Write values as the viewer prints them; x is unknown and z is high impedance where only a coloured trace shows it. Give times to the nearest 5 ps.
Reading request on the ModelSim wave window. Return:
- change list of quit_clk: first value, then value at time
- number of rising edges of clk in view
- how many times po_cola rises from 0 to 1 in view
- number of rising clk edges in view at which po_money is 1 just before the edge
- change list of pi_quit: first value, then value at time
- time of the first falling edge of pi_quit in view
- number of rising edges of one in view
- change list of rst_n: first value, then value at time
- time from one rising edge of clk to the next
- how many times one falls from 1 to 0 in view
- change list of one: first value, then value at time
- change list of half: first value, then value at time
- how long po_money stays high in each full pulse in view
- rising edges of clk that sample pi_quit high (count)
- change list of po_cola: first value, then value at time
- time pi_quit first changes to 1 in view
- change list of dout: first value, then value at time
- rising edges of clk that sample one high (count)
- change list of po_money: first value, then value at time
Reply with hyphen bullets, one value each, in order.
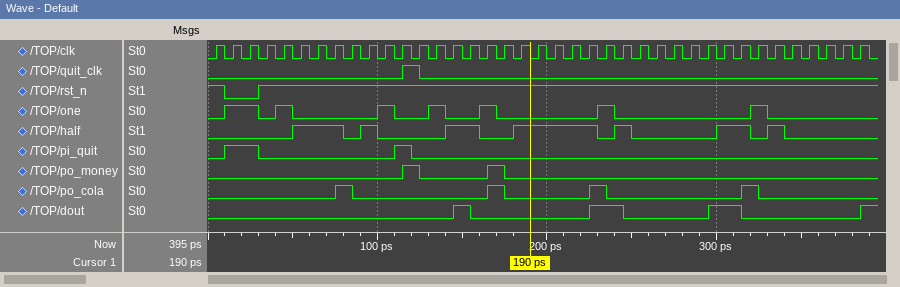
- 0, 1 at 115 ps, 0 at 125 ps
- 39
- 4
- 2
- 0, 1 at 10 ps, 0 at 30 ps, 1 at 110 ps, 0 at 120 ps
- 30 ps
- 7
- 1, 0 at 10 ps, 1 at 30 ps
- 10 ps
- 7
- 0, 1 at 10 ps, 0 at 30 ps, 1 at 40 ps, 0 at 50 ps, 1 at 100 ps, 0 at 110 ps, 1 at 130 ps, 0 at 140 ps, 1 at 160 ps, 0 at 170 ps, 1 at 230 ps, 0 at 240 ps, 1 at 320 ps, 0 at 330 ps
- 0, 1 at 50 ps, 0 at 80 ps, 1 at 90 ps, 0 at 100 ps, 1 at 140 ps, 0 at 160 ps, 1 at 180 ps, 0 at 230 ps, 1 at 240 ps, 0 at 250 ps, 1 at 300 ps, 0 at 320 ps, 1 at 330 ps, 0 at 340 ps
- 10 ps, 10 ps
- 3
- 0, 1 at 75 ps, 0 at 85 ps, 1 at 165 ps, 0 at 175 ps, 1 at 225 ps, 0 at 235 ps, 1 at 315 ps, 0 at 325 ps
- 10 ps
- 0, 1 at 145 ps, 0 at 155 ps, 1 at 225 ps, 0 at 245 ps, 1 at 295 ps, 0 at 315 ps, 1 at 385 ps
- 8
- 0, 1 at 115 ps, 0 at 125 ps, 1 at 165 ps, 0 at 175 ps
